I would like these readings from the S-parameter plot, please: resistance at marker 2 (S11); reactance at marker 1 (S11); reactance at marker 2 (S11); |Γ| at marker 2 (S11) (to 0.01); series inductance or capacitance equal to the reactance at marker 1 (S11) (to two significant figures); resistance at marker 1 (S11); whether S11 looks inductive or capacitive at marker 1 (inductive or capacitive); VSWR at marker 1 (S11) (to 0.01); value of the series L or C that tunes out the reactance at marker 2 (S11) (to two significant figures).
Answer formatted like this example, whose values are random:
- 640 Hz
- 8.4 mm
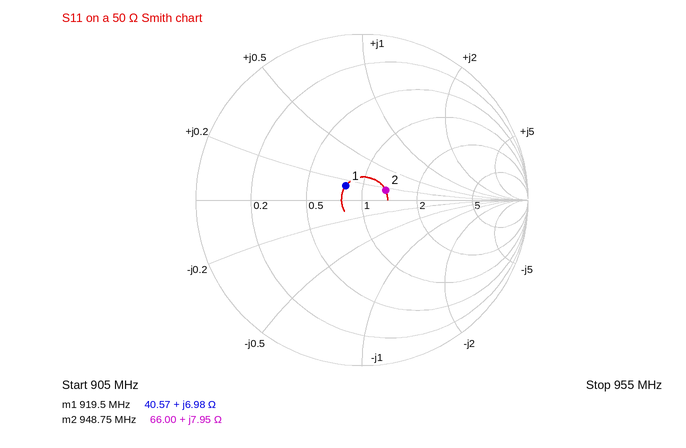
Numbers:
- 66.00 Ω
- +6.98 Ω
- +7.95 Ω
- 0.15
- 1.2 nH
- 40.57 Ω
- inductive
- 1.30
- 21 pF
